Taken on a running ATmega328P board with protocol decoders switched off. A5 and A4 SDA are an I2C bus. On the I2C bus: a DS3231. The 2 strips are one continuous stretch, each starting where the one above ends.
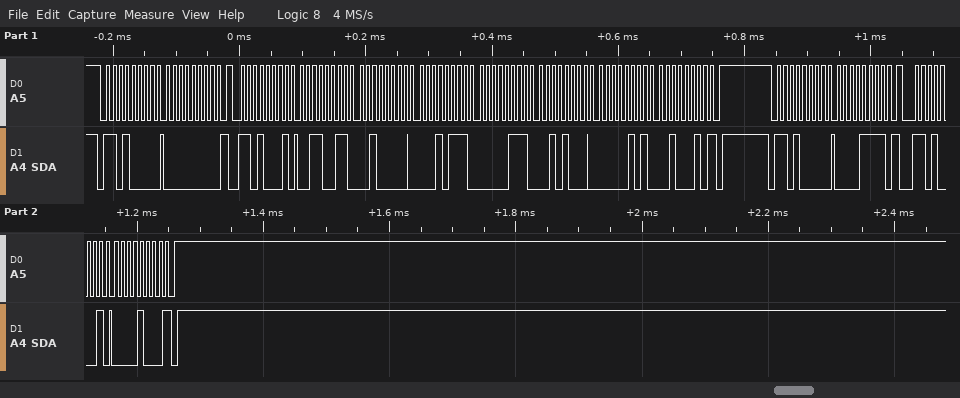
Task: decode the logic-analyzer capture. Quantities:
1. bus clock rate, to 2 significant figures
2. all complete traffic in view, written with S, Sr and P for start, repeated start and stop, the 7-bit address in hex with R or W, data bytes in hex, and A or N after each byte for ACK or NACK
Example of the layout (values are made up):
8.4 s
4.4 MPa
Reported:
100 kHz
S 68W A 00 A Sr 68R A 33 A 20 A 17 A 07 A 28 A 05 A 22 N P S 68W A 0F A Sr 68R A 08 N P
